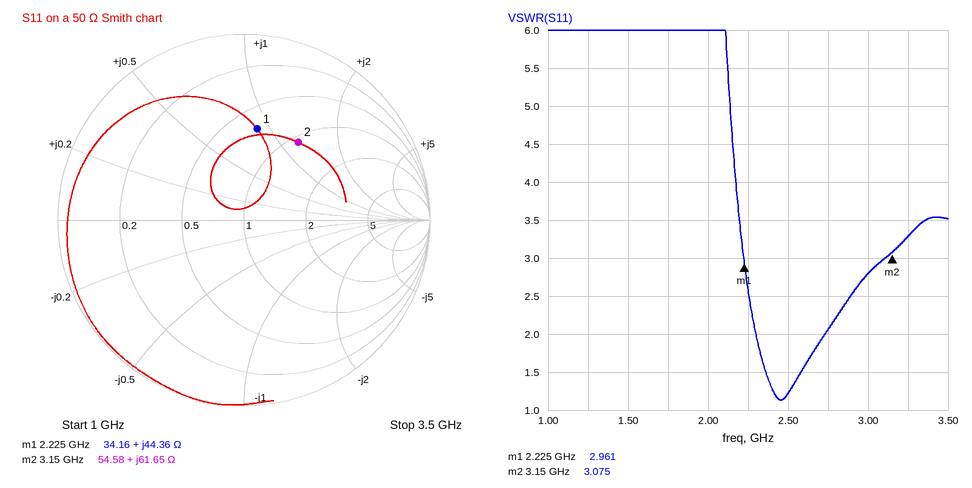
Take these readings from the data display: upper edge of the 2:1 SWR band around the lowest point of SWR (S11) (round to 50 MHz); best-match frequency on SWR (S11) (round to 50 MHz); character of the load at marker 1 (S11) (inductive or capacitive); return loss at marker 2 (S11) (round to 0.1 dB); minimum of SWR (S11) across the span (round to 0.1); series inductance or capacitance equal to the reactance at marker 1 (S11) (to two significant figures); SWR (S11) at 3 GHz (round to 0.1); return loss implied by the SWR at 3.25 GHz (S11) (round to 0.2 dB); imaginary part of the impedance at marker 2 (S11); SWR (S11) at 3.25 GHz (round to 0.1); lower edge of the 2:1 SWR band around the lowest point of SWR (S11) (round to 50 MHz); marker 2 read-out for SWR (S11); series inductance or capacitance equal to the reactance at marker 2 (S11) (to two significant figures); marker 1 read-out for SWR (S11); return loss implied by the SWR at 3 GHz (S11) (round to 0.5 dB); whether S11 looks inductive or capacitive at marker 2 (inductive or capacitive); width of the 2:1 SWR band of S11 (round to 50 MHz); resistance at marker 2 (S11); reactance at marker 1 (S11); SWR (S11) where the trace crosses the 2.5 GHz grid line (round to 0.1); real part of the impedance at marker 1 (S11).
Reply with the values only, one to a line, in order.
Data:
2.75 GHz
2.45 GHz
inductive
5.9 dB
1.1
3.2 nH
2.8
5.4 dB
+61.65 Ω
3.3
2.30 GHz
3.075
3.1 nH
2.961
6.5 dB
inductive
450 MHz
54.58 Ω
+44.36 Ω
1.2
34.16 Ω
